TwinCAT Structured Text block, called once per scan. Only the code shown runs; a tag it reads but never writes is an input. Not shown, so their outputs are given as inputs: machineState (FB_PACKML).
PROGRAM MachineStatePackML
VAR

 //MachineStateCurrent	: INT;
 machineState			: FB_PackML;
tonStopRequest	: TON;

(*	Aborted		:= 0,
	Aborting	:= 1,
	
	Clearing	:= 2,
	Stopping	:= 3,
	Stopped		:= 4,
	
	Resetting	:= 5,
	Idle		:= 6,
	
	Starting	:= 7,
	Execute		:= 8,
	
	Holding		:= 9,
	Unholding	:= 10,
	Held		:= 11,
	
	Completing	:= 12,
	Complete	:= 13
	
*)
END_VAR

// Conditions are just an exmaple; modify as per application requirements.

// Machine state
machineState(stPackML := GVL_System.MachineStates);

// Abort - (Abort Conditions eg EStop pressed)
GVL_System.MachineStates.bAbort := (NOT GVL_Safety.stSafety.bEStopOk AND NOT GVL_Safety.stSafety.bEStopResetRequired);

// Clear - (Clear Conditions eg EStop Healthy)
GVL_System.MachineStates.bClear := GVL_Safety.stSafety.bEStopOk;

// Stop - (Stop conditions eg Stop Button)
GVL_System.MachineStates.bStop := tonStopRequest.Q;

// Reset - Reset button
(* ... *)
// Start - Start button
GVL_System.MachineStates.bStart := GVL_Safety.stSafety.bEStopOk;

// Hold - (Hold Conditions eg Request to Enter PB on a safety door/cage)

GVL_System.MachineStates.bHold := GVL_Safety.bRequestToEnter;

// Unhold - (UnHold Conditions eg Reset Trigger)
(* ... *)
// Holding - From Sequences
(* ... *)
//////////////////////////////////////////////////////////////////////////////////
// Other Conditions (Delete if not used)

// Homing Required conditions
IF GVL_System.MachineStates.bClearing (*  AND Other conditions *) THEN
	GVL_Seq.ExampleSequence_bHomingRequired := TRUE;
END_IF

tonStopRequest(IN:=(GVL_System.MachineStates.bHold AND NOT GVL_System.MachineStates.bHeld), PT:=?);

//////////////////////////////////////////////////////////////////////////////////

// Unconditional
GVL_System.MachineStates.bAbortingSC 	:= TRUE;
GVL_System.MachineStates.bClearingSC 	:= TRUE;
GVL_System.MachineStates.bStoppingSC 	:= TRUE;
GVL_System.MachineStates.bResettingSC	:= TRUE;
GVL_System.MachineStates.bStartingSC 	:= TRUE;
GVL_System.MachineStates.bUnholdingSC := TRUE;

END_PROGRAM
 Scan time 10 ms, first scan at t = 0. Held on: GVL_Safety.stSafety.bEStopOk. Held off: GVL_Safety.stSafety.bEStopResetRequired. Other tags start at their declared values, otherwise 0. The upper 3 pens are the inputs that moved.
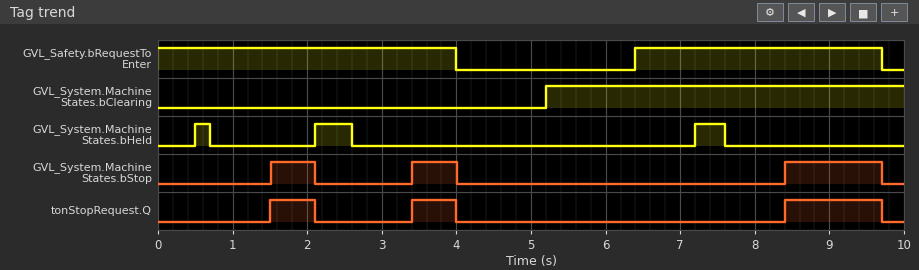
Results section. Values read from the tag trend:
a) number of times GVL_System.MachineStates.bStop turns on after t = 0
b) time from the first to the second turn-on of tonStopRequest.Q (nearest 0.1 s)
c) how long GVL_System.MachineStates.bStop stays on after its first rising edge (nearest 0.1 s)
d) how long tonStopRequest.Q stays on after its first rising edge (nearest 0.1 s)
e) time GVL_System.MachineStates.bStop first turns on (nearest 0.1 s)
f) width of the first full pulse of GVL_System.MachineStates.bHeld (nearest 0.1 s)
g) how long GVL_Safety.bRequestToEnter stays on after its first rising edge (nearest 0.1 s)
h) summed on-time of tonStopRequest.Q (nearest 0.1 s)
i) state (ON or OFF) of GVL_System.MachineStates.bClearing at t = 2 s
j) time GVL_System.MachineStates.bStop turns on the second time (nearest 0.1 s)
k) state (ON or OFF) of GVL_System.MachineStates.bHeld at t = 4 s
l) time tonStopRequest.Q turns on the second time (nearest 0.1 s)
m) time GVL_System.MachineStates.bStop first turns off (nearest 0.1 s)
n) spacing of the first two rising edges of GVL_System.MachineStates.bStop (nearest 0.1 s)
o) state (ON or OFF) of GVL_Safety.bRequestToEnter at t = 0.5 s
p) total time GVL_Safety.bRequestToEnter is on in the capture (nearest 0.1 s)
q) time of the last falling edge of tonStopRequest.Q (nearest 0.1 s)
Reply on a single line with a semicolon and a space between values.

3; 1.9 s; 0.6 s; 0.6 s; 1.5 s; 0.2 s; 3.3 s; 2.5 s; OFF; 3.4 s; OFF; 3.4 s; 2.1 s; 1.9 s; ON; 7.3 s; 9.7 s
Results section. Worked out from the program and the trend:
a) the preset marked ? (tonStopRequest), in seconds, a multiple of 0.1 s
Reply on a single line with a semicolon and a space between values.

0.8 s
